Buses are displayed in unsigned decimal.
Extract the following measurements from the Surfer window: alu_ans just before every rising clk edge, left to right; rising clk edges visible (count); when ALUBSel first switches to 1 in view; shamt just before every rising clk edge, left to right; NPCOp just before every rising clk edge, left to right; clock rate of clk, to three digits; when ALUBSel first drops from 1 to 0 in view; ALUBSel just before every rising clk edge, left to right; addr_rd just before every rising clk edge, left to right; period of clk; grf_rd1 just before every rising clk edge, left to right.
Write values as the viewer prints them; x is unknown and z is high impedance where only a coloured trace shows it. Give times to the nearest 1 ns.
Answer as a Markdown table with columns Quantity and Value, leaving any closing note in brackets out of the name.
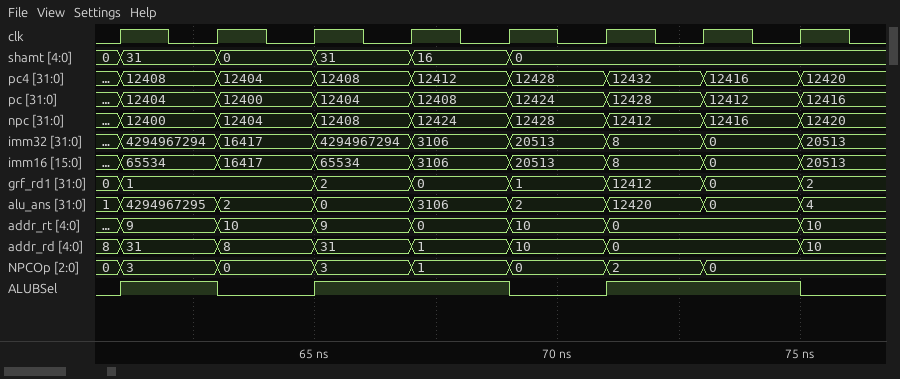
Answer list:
| Quantity | Value |
|---|---|
| alu_ans just before every rising clk edge, left to right | 1, 4294967295, 2, 0, 3106, 2, 12420, 0 |
| rising clk edges visible | 8 |
| when ALUBSel first switches to 1 in view | 61 ns |
| shamt just before every rising clk edge, left to right | 0, 31, 0, 31, 16, 0, 0, 0 |
| NPCOp just before every rising clk edge, left to right | 0, 3, 0, 3, 1, 0, 2, 0 |
| clock rate of clk, to three digits | 500 MHz |
| when ALUBSel first drops from 1 to 0 in view | 63 ns |
| ALUBSel just before every rising clk edge, left to right | 0 1 0 1 1 0 1 1 |
| addr_rd just before every rising clk edge, left to right | 8, 31, 8, 31, 1, 10, 0, 0 |
| period of clk | 2 ns |
| grf_rd1 just before every rising clk edge, left to right | 0, 1, 1, 2, 0, 1, 12412, 0 |
